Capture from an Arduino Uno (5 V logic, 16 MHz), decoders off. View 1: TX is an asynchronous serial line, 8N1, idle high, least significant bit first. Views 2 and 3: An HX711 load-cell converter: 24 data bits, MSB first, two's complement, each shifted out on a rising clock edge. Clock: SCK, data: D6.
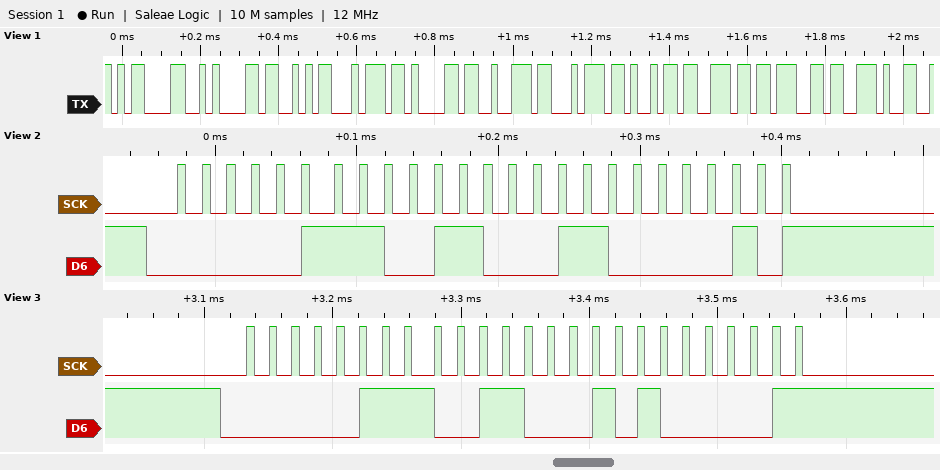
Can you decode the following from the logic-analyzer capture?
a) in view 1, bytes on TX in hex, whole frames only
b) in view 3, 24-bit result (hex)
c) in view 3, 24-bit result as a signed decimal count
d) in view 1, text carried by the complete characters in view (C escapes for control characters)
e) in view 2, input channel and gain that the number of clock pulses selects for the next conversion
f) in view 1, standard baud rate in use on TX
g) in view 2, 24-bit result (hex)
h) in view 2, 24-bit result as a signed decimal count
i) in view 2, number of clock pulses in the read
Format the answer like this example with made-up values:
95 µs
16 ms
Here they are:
0D 0A 53 74 61 72 74 69 6E 67 2E
0x073141
471361
"\r\nStarting."
channel A, gain 128
57600 baud
0x073182
471426
25
